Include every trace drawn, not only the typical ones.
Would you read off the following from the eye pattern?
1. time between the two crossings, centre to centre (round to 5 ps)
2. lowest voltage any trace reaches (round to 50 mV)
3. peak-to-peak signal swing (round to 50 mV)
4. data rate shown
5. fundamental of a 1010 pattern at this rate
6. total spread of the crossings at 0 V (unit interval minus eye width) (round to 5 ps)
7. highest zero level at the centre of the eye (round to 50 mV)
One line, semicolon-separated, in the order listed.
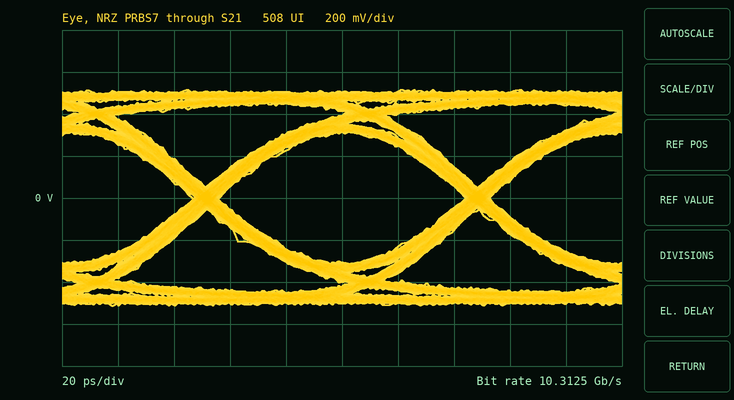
95 ps; -500 mV; 1.05 V; 10.3125 Gb/s; 5.15625 GHz; 10 ps; -300 mV
